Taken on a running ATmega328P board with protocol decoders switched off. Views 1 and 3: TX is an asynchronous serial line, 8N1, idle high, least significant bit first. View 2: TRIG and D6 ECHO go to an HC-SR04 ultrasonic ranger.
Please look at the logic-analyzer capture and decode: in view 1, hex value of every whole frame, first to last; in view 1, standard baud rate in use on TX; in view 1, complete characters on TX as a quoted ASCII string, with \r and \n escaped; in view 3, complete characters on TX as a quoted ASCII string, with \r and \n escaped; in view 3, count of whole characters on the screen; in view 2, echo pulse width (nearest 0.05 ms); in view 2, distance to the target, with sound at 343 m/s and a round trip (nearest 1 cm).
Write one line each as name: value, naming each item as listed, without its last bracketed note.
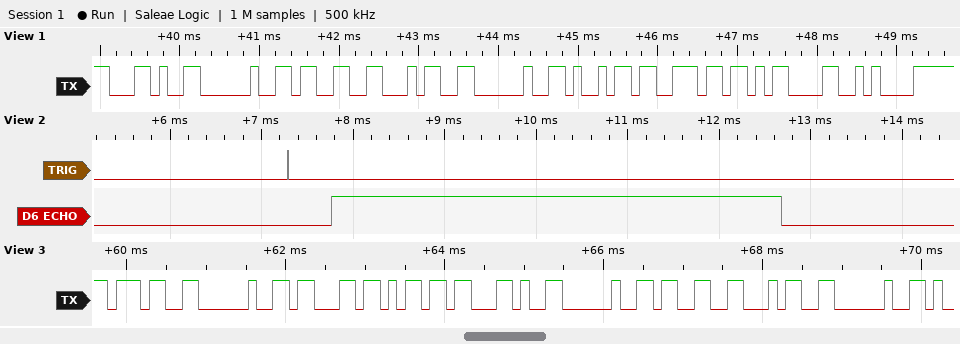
in view 1, hex value of every whole frame, first to last: 2C 20 33 34 20 69 6E 0D 0A
in view 1, standard baud rate in use on TX: 9600 baud
in view 1, complete characters on TX as a quoted ASCII string, with \r and \n escaped: ", 34 in\r\n"
in view 3, complete characters on TX as a quoted ASCII string, with \r and \n escaped: "7 cm, 34 "
in view 3, count of whole characters on the screen: 9
in view 2, echo pulse width: 4.90 ms
in view 2, distance to the target, with sound at 343 m/s and a round trip: 84 cm
